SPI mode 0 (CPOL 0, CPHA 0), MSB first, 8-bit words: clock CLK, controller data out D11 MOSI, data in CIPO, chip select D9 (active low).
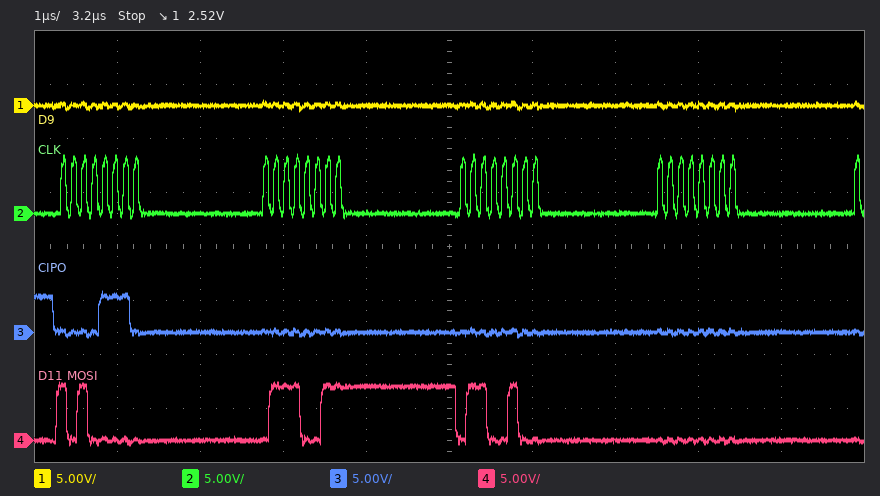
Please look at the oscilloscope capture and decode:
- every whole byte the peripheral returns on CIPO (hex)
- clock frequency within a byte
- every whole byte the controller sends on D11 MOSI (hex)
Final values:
0E 00 00 00
8 MHz
A0 73 64 00
